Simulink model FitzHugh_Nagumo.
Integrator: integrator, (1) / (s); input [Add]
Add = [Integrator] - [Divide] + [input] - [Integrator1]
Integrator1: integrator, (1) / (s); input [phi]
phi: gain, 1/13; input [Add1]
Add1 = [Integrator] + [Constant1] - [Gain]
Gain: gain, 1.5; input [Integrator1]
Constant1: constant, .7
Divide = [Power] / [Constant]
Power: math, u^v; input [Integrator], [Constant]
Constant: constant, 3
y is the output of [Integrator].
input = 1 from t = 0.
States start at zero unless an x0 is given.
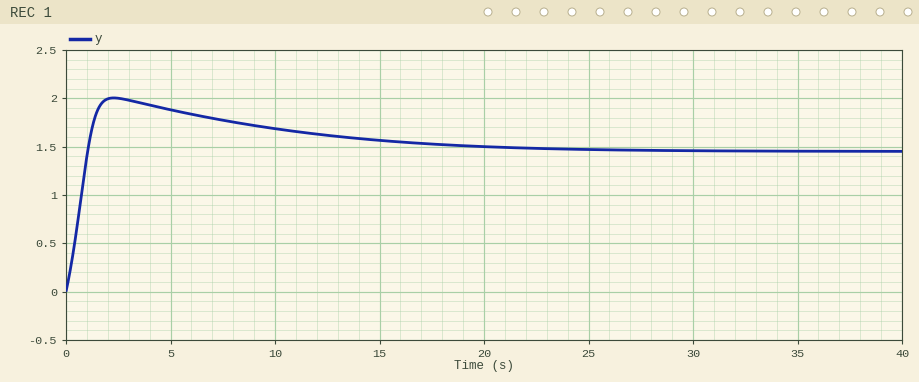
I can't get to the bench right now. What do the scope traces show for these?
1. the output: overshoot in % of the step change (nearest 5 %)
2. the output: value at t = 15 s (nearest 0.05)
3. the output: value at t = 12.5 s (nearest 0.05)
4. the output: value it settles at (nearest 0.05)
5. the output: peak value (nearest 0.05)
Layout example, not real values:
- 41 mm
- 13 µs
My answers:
- 40 %
- 1.55
- 1.60
- 1.45
- 2.00
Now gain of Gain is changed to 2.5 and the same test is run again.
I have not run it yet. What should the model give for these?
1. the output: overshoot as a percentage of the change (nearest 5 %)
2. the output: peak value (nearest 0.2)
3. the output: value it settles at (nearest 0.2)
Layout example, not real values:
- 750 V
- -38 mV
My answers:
- 15 %
- 2.0
- 1.8
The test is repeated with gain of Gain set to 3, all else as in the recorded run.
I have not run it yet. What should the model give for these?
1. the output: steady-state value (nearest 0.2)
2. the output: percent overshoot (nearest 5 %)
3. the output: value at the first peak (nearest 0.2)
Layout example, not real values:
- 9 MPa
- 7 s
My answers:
- 1.8
- 10 %
- 2.0
